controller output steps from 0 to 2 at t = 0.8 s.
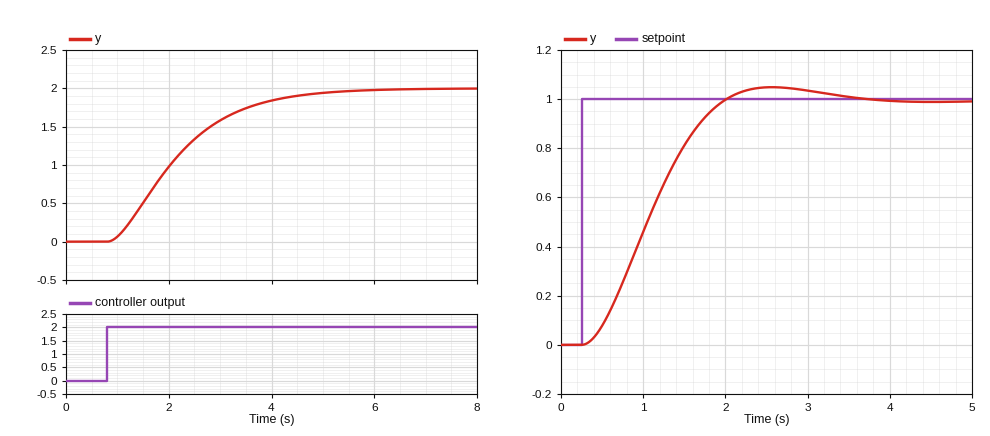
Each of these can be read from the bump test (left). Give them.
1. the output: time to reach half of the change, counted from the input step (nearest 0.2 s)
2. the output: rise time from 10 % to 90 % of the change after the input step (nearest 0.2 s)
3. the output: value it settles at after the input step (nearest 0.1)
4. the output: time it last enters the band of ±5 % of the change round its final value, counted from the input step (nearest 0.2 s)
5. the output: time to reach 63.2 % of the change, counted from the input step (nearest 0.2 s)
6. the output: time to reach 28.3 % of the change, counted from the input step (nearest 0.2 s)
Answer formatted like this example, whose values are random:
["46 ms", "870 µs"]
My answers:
["1.2 s", "2.6 s", "2.0", "3.6 s", "1.6 s", "0.8 s"]
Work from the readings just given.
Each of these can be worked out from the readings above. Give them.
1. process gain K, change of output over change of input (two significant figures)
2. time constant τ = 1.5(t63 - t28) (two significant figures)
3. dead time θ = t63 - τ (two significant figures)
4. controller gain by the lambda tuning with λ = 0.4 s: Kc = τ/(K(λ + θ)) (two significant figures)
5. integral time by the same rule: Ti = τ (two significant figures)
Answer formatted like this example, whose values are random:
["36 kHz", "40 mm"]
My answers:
["1.0", "1.2 s", "0.40 s", "1.5", "1.2 s"]
